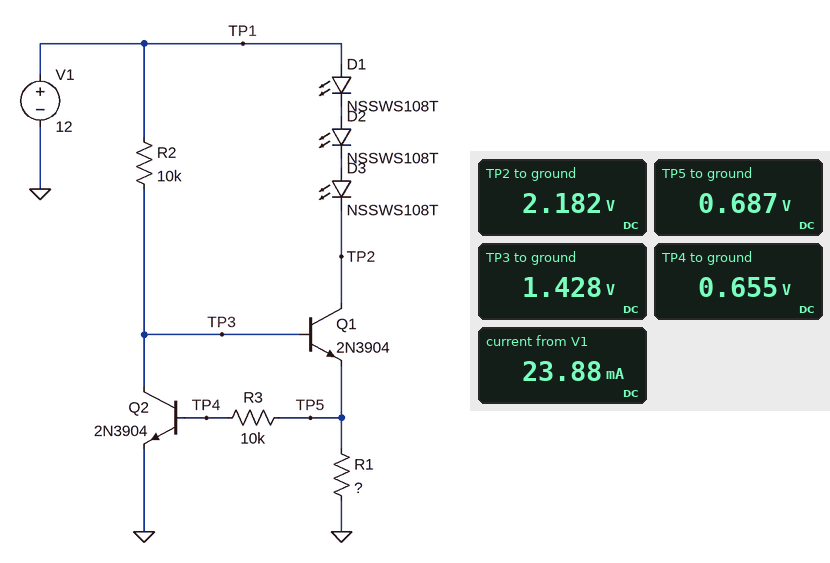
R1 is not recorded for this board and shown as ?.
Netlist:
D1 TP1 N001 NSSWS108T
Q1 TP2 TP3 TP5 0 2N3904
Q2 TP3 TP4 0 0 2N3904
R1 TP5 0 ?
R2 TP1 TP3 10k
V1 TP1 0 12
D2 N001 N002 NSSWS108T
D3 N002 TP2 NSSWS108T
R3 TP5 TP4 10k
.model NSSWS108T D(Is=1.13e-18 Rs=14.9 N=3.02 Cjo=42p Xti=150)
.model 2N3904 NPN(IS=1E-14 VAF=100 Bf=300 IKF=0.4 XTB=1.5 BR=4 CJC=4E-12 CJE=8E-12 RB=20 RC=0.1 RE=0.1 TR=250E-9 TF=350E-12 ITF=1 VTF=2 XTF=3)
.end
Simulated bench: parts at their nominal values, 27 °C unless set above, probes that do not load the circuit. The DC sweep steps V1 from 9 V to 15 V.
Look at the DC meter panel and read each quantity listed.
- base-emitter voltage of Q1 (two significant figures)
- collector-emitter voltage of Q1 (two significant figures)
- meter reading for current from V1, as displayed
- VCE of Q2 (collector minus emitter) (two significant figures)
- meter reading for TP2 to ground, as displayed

740 mV
1.5 V
23.88 mA
1.4 V
2.182 V
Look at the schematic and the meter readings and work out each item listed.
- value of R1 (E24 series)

30 Ω
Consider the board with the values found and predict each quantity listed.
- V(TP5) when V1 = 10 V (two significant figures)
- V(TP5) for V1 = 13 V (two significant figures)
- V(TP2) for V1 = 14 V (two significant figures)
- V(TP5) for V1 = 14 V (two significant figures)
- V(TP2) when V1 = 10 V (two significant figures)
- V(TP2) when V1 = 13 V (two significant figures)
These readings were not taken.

510 mV
690 mV
4.2 V
700 mV
560 mV
3.2 V
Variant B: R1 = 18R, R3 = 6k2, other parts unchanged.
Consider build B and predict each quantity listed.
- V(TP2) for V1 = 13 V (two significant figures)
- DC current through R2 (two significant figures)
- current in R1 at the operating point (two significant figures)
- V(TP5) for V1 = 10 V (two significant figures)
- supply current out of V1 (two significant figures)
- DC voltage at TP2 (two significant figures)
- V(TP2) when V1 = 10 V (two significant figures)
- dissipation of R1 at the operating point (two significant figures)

2.4 V
1.1 mA
37 mA
350 mV
38 mA
1.4 V
410 mV
25 mW
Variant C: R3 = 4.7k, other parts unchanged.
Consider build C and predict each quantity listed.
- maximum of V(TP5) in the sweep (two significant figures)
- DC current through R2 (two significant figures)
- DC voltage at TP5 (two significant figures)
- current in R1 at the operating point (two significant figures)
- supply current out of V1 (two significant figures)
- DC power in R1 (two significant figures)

680 mV
1.1 mA
670 mV
22 mA
23 mA
15 mW
